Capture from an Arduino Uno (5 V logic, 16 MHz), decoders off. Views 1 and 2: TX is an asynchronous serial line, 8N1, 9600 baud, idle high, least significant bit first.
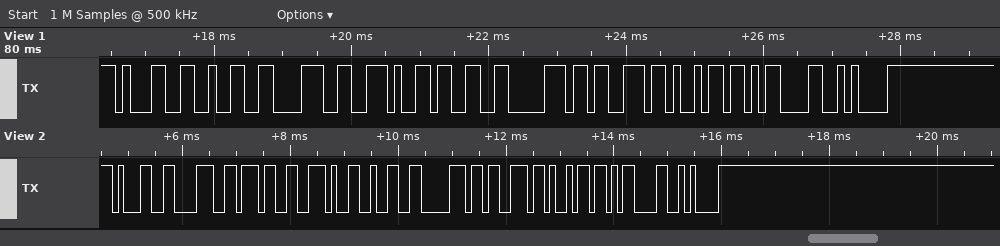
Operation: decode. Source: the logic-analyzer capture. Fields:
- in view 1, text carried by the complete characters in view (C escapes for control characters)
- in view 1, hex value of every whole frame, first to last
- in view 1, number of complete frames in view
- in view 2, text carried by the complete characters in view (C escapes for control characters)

"128.3psi\r\n"
0x31 0x32 0x38 0x2E 0x33 0x70 0x73 0x69 0x0D 0x0A
10
"187.2psi\r\n"
